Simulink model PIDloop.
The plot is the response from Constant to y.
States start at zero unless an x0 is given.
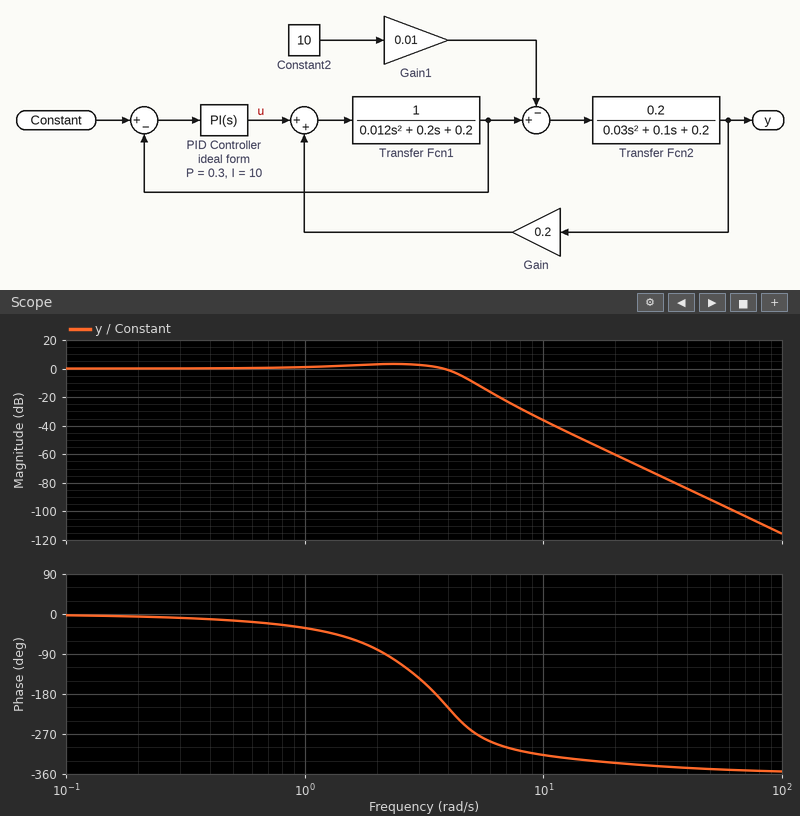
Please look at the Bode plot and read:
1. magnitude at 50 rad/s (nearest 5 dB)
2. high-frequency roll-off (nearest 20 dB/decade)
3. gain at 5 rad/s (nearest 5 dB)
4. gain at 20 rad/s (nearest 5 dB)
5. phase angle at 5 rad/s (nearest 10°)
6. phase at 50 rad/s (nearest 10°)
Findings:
-90 dB
-80 dB/decade
-10 dB
-60 dB
-260°
-350°
